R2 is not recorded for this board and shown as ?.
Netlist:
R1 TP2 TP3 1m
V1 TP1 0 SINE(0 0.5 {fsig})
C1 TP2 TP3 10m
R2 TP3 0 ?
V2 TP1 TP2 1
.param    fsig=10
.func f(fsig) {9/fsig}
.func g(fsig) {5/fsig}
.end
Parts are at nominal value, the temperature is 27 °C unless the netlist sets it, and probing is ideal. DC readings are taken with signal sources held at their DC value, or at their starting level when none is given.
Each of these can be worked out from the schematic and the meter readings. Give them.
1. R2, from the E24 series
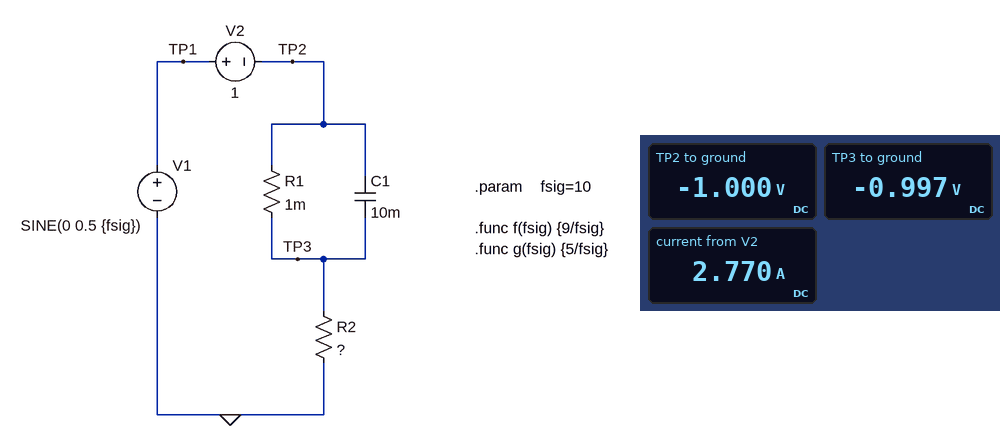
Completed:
0.36 Ω
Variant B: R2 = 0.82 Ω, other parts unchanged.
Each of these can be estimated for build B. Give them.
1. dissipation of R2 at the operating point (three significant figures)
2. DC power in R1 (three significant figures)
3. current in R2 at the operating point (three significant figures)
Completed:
1.22 W
1.48 mW
1.22 A
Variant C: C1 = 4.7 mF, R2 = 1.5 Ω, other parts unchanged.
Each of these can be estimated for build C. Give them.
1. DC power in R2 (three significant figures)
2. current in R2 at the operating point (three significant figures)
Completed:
666 mW
666 mA
